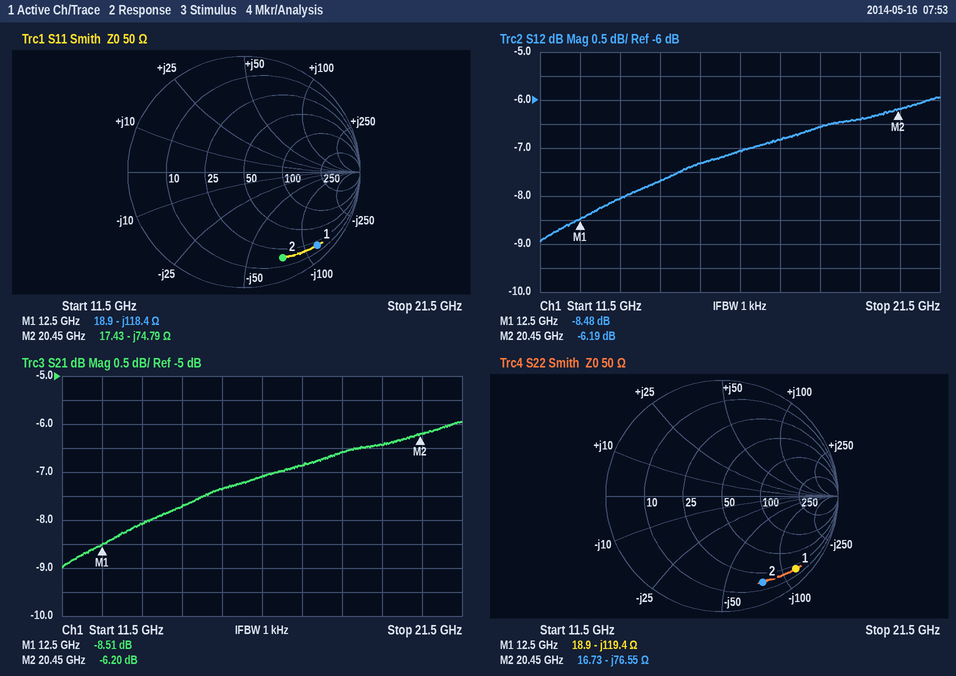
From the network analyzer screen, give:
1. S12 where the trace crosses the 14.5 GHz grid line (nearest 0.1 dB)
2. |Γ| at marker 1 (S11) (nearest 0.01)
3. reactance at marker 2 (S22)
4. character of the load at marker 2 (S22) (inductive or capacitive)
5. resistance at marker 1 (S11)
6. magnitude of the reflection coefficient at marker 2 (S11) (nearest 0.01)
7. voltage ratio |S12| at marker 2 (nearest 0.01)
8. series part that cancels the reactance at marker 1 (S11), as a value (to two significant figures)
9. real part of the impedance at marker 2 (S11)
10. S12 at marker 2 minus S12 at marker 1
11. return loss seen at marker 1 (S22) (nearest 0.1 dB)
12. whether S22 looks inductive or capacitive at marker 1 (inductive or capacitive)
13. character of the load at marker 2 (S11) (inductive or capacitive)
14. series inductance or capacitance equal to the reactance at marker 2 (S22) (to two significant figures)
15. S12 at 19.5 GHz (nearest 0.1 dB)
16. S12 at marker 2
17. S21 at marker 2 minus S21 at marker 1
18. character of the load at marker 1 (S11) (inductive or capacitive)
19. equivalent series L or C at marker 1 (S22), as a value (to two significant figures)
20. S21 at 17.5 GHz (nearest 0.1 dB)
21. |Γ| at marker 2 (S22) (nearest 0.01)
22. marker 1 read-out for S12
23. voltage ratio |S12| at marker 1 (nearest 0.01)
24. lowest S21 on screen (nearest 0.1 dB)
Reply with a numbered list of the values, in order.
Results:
1. -7.7 dB
2. 0.89
3. -76.55 Ω
4. capacitive
5. 18.9 Ω
6. 0.81
7. 0.49
8. 1.5 nH
9. 17.43 Ω
10. 2.29 dB
11. 1.0 dB
12. capacitive
13. capacitive
14. 100 fF
15. -6.4 dB
16. -6.19 dB
17. 2.31 dB
18. capacitive
19. 110 fF
20. -6.9 dB
21. 0.82
22. -8.48 dB
23. 0.38
24. -9.0 dB
